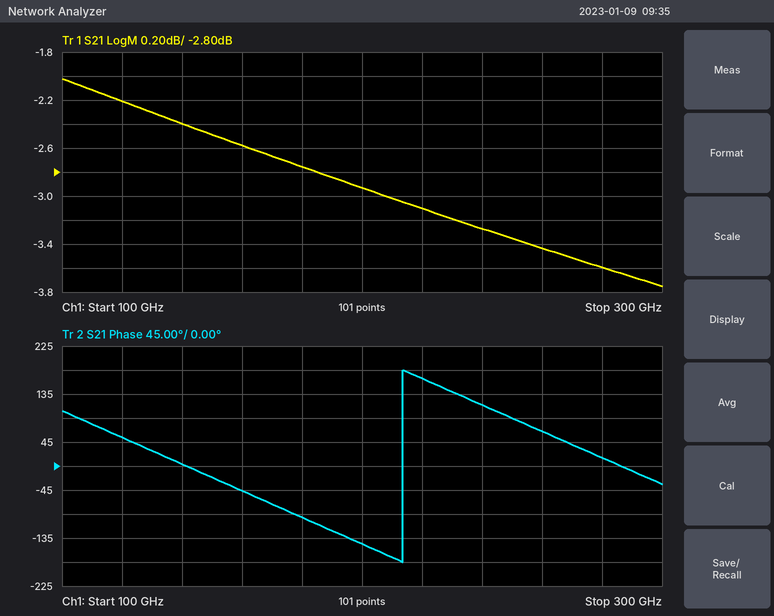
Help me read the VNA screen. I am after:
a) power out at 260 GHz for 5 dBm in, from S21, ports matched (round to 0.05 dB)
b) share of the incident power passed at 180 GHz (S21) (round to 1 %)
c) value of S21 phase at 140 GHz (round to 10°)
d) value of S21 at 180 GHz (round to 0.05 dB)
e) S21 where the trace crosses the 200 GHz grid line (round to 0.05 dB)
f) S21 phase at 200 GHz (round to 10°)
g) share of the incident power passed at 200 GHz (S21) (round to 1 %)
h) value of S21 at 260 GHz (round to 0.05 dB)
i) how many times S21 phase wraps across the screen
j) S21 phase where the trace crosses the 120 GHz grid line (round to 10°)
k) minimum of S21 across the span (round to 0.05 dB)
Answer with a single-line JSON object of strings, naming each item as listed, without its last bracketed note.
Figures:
{"power out at 260 GHz for 5 dBm in, from S21, ports matched": "1.55 dBm", "share of the incident power passed at 180 GHz (S21)": "53 %", "value of S21 phase at 140 GHz": "0°", "value of S21 at 180 GHz": "-2.75 dB", "S21 where the trace crosses the 200 GHz grid line": "-2.95 dB", "S21 phase at 200 GHz": "-150°", "share of the incident power passed at 200 GHz (S21)": "51 %", "value of S21 at 260 GHz": "-3.45 dB", "how many times S21 phase wraps across the screen": "1", "S21 phase where the trace crosses the 120 GHz grid line": "50°", "minimum of S21 across the span": "-3.75 dB"}
